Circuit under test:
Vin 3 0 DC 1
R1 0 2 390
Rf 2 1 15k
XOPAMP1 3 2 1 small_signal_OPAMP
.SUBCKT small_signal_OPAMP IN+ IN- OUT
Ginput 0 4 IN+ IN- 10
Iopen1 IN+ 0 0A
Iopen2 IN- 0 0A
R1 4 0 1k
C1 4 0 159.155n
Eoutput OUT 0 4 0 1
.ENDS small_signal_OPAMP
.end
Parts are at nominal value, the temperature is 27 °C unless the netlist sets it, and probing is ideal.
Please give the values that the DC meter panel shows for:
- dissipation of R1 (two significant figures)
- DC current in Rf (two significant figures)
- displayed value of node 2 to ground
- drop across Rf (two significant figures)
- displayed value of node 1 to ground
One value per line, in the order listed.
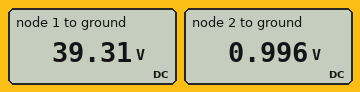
2.5 mW
2.6 mA
0.996 V
38 V
39.31 V
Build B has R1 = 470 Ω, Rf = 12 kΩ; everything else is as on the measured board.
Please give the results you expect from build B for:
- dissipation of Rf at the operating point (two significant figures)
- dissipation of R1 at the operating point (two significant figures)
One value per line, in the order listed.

54 mW
2.1 mW
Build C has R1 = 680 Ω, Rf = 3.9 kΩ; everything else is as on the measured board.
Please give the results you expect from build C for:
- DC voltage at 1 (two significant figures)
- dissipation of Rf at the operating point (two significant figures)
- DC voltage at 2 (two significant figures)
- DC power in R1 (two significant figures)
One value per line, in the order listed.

6.7 V
8.4 mW
1.0 V
1.5 mW
